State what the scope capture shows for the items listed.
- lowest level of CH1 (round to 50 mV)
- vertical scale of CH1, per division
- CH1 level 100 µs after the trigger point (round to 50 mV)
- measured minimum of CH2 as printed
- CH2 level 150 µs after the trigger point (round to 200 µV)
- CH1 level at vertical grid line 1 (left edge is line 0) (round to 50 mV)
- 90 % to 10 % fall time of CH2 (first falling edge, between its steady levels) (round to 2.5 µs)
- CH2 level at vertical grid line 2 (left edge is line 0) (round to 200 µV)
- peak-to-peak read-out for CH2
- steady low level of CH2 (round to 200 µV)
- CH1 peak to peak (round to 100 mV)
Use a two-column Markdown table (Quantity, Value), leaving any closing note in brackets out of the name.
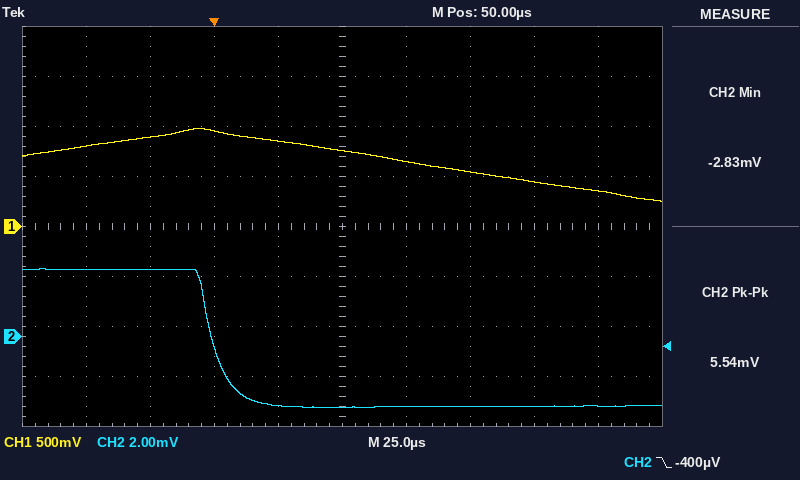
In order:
| Quantity | Value |
|---|---|
| lowest level of CH1 | 250 mV |
| vertical scale of CH1, per division | 500 mV |
| CH1 level 100 µs after the trigger point | 550 mV |
| measured minimum of CH2 as printed | -2.83 mV |
| CH2 level 150 µs after the trigger point | -2.8 mV |
| CH1 level at vertical grid line 1 (left edge is line 0) | 800 mV |
| 90 % to 10 % fall time of CH2 (first falling edge, between its steady levels) | 15.0 µs |
| CH2 level at vertical grid line 2 (left edge is line 0) | 2.6 mV |
| peak-to-peak read-out for CH2 | 5.54 mV |
| steady low level of CH2 | -2.8 mV |
| CH1 peak to peak | 700 mV |
